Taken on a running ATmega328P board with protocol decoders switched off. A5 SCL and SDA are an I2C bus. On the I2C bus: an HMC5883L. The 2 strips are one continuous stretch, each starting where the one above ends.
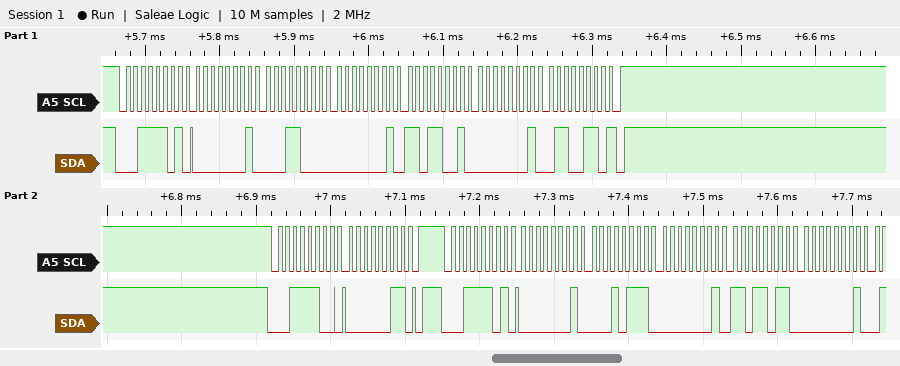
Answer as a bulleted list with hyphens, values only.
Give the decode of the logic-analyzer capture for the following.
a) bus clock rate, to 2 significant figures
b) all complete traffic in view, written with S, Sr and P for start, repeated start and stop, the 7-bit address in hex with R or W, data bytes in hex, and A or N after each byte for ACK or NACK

- 100 kHz
- S 1ER A 01 A 18 A 01 A D9 A 01 A 66 N P S 1EW A 03 A P S 1ER A 01 A 17 A 01 A DB A 01 A
